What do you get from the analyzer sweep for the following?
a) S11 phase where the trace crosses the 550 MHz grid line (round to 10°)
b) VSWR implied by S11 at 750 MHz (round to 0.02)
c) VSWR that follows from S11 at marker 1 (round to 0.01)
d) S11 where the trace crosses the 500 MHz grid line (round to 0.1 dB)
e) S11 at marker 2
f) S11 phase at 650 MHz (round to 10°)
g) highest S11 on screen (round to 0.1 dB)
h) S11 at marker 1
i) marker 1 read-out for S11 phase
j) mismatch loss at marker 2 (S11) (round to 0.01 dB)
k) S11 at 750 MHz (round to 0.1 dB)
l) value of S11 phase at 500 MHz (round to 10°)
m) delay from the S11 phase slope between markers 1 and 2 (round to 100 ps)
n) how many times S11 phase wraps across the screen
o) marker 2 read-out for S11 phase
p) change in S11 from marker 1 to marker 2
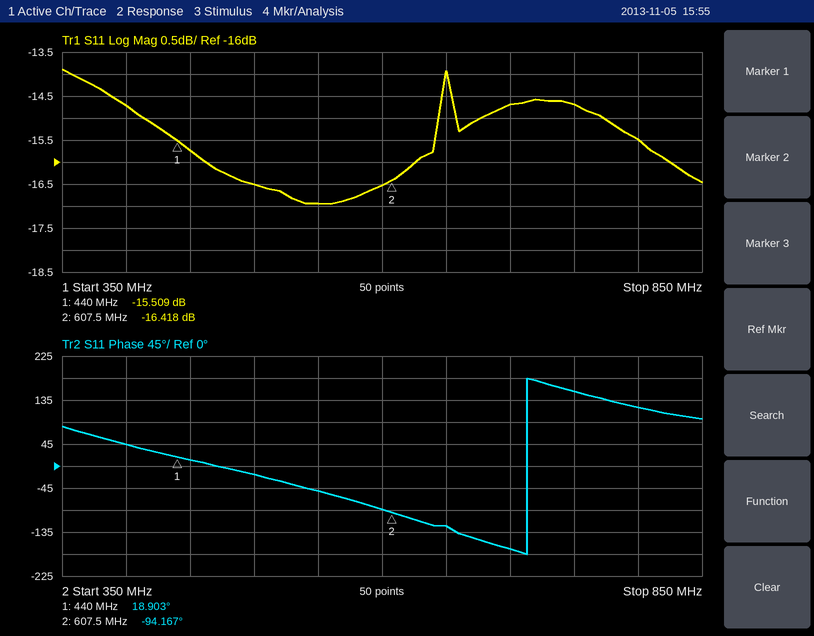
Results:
-50°
1.46
1.40
-16.5 dB
-16.418 dB
-120°
-13.9 dB
-15.509 dB
18.903°
0.10 dB
-14.7 dB
-20°
1.9 ns
1
-94.167°
-0.909 dB
